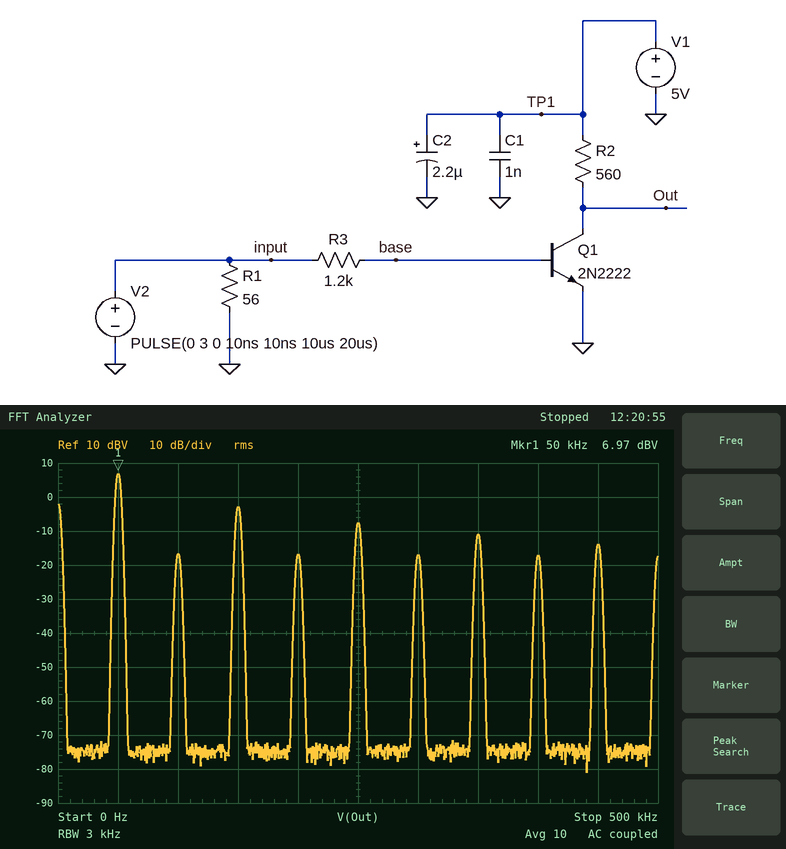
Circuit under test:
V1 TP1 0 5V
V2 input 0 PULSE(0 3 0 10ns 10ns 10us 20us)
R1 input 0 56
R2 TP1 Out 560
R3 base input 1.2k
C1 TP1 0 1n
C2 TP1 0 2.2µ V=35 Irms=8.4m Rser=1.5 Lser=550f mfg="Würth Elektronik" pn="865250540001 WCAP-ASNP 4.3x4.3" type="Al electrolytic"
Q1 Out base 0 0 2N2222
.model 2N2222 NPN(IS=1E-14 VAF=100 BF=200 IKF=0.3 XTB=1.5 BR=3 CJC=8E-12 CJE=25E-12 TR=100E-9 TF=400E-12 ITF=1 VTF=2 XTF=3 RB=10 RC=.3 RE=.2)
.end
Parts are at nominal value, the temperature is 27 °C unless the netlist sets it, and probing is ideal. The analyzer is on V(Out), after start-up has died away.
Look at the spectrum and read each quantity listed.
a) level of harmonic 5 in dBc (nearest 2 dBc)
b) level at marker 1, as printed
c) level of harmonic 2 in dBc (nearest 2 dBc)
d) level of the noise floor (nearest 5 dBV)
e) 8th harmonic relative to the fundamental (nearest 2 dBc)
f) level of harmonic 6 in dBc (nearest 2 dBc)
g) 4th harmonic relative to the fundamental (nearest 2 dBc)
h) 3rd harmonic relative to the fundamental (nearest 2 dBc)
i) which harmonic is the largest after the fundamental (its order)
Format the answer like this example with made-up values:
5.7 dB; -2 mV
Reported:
-14 dBc; 6.97 dBV; -24 dBc; -75 dBV; -24 dBc; -24 dBc; -24 dBc; -10 dBc; 3
